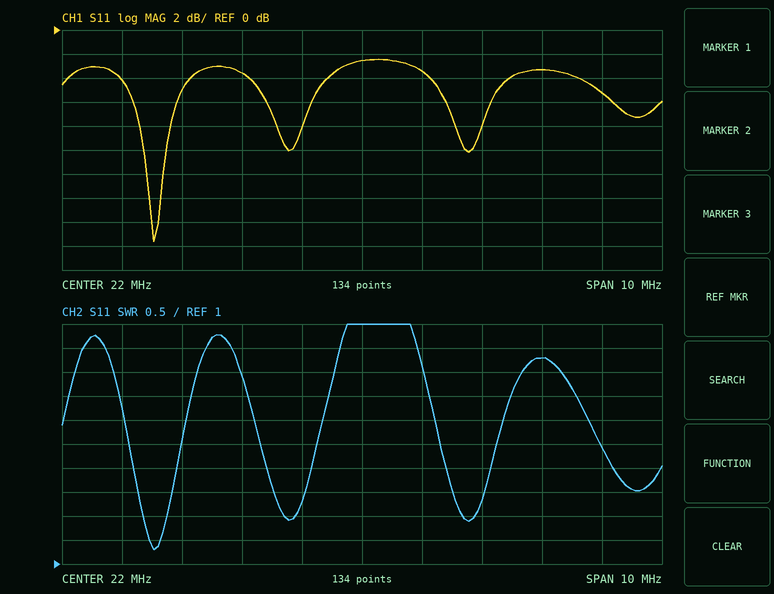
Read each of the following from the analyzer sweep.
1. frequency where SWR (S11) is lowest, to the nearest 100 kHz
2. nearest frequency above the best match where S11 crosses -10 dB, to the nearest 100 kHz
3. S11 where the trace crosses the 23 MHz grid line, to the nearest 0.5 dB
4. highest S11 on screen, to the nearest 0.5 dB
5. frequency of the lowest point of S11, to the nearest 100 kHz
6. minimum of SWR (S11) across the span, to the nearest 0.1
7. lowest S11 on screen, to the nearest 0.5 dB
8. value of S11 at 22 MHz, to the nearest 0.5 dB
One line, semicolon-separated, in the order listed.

18.5 MHz; 18.7 MHz; -3.5 dB; -2.5 dB; 18.5 MHz; 1.3; -17.5 dB; -2.5 dB
